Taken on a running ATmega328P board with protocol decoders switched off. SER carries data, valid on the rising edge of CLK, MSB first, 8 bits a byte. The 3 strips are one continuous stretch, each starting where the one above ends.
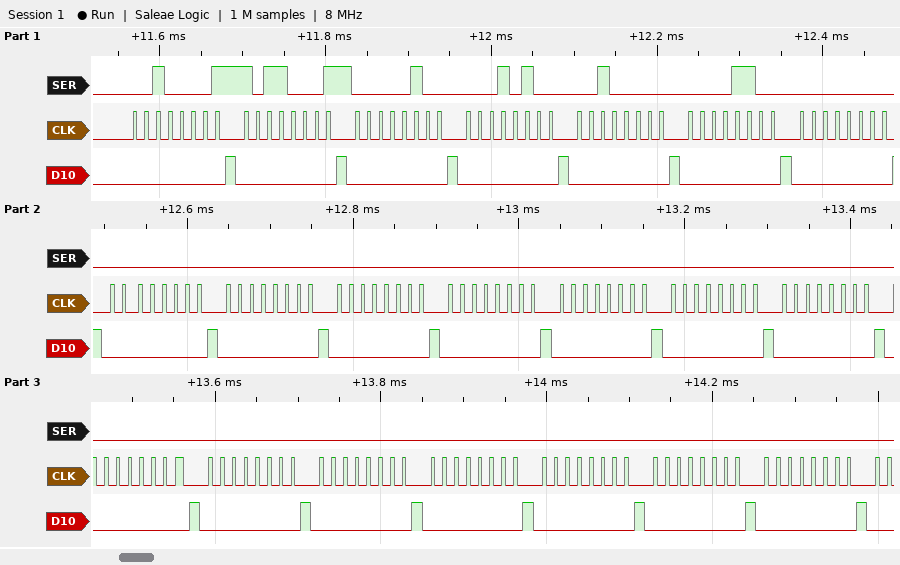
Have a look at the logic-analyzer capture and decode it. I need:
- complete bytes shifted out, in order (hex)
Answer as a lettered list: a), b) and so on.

a) 21 B1 04 14 20 0C 00 00 00 00 00 00 00 00 00 00 00 00 00 00 00
